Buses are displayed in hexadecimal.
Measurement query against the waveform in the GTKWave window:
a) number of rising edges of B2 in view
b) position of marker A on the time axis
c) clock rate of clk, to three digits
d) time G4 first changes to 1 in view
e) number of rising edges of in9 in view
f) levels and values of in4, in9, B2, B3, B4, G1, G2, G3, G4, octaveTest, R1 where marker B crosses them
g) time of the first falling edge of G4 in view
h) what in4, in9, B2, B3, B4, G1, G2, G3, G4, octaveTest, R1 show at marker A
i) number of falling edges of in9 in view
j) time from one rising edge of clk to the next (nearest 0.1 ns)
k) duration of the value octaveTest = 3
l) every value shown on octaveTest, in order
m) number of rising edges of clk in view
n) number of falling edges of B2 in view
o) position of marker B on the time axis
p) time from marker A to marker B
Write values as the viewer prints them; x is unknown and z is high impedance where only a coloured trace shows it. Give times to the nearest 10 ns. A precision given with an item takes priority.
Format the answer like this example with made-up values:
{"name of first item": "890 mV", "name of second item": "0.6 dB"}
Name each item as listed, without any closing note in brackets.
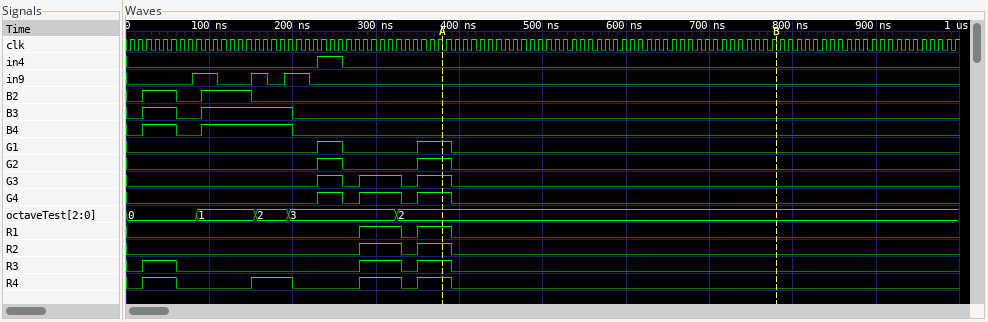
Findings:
{"number of rising edges of B2 in view": "2", "position of marker A on the time axis": "380 ns", "clock rate of clk, to three digits": "100 MHz", "time G4 first changes to 1 in view": "230 ns", "number of rising edges of in9 in view": "3", "levels and values of in4, in9, B2, B3, B4, G1, G2, G3, G4, octaveTest, R1 where marker B crosses them": "in4=0, in9=0, B2=0, B3=0, B4=0, G1=0, G2=0, G3=0, G4=0, octaveTest=2, R1=0", "time of the first falling edge of G4 in view": "260 ns", "what in4, in9, B2, B3, B4, G1, G2, G3, G4, octaveTest, R1 show at marker A": "in4=0, in9=0, B2=0, B3=0, B4=0, G1=1, G2=1, G3=1, G4=1, octaveTest=2, R1=1", "number of falling edges of in9 in view": "3", "time from one rising edge of clk to the next": "10 ns", "duration of the value octaveTest = 3": "130 ns", "every value shown on octaveTest, in order": "0, 1, 2, 3, 2", "number of rising edges of clk in view": "100", "number of falling edges of B2 in view": "2", "position of marker B on the time axis": "780 ns", "time from marker A to marker B": "400 ns"}
